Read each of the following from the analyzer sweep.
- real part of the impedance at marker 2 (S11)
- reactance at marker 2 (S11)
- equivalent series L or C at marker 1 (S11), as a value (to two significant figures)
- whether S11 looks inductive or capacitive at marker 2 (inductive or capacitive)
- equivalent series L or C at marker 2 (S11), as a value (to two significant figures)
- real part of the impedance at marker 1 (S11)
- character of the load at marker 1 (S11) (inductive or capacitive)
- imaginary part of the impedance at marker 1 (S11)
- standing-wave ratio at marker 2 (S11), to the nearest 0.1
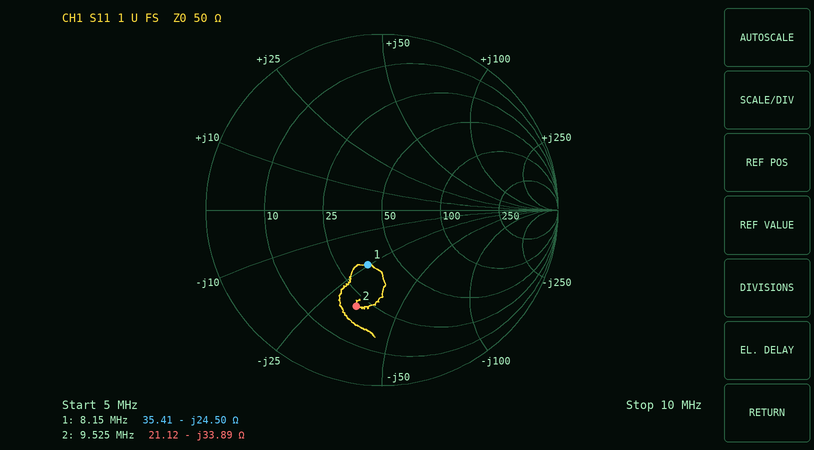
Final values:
21.12 Ω
-33.89 Ω
800 pF
capacitive
490 pF
35.41 Ω
capacitive
-24.50 Ω
3.6
